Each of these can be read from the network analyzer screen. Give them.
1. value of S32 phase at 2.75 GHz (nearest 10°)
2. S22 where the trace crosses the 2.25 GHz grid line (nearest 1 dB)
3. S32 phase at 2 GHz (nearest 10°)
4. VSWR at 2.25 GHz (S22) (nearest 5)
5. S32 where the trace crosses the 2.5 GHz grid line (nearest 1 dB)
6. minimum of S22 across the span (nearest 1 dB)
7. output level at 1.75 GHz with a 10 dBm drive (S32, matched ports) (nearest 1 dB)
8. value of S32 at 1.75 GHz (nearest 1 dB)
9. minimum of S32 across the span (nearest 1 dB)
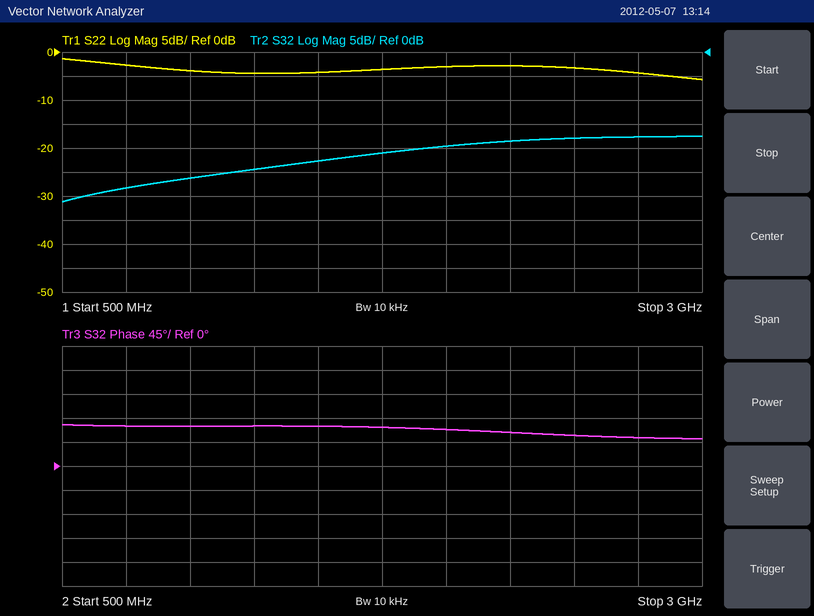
50°
-3 dB
70°
5
-18 dB
-6 dB
-11 dBm
-21 dB
-31 dB
